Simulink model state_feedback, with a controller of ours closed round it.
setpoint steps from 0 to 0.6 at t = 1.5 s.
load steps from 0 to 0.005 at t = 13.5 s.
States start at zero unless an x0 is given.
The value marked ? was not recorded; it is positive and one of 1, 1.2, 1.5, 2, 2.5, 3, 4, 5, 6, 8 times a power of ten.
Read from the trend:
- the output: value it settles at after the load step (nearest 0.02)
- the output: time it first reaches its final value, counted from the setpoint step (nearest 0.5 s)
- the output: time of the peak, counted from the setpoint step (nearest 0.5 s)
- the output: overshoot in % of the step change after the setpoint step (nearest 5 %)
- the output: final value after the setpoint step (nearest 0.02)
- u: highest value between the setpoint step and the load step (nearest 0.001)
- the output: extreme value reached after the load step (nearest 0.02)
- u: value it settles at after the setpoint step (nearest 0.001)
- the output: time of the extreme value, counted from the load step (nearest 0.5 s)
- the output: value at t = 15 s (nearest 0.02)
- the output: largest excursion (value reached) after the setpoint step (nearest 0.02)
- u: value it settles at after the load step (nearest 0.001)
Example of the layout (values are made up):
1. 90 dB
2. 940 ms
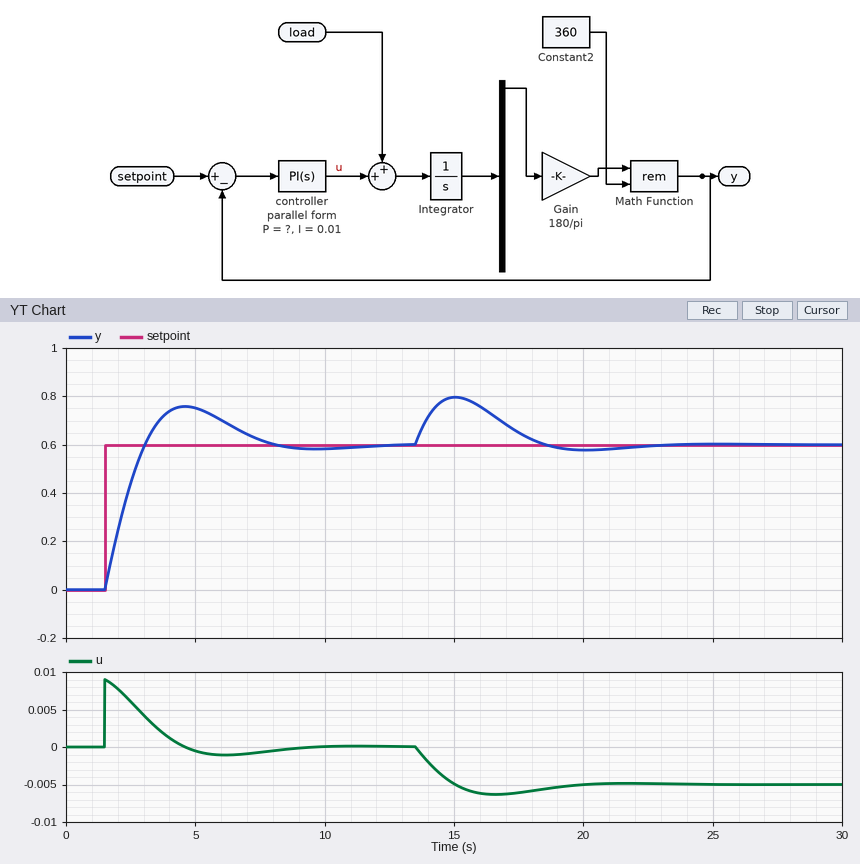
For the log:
1. 0.60
2. 1.5 s
3. 3.0 s
4. 25 %
5. 0.60
6. 0.009
7. 0.80
8. 0.000
9. 1.5 s
10. 0.80
11. 0.76
12. -0.005
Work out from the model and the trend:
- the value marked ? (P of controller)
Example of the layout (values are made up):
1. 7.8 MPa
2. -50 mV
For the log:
1. 0.015
